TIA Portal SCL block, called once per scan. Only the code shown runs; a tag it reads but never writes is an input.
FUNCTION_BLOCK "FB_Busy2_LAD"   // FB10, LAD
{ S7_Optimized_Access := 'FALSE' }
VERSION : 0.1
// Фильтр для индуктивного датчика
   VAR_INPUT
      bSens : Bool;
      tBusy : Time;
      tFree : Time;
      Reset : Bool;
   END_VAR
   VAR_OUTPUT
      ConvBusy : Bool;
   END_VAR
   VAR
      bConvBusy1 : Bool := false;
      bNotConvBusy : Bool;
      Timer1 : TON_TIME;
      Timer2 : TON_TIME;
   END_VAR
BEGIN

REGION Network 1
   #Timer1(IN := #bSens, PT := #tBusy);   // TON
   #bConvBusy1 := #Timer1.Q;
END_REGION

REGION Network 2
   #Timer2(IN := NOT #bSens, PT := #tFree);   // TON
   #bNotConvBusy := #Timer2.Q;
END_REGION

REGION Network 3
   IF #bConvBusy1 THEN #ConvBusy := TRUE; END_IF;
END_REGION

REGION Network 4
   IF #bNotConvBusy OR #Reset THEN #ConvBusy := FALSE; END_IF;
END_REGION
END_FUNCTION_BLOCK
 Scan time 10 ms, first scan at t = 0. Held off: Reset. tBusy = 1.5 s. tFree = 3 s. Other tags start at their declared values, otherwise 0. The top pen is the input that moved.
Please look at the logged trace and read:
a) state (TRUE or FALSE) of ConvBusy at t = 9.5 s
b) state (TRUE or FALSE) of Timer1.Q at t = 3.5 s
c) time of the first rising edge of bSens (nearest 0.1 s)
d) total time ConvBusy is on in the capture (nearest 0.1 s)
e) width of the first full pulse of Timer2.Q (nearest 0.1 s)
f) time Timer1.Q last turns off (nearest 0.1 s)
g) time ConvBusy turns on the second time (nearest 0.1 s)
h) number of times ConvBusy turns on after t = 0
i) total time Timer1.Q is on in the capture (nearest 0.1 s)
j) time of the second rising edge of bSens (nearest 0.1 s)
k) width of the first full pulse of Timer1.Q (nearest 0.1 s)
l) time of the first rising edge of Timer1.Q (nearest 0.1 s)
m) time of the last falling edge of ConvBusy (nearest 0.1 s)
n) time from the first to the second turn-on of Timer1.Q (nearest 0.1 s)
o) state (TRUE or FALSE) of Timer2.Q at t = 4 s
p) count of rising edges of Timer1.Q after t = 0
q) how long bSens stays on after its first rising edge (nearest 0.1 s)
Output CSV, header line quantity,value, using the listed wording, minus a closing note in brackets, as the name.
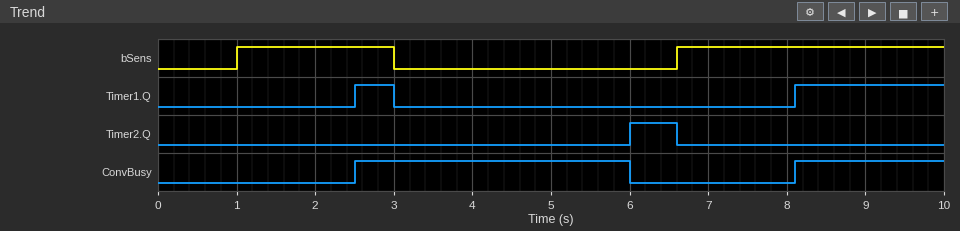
quantity,value
state (TRUE or FALSE) of ConvBusy at t = 9.5 s,TRUE
state (TRUE or FALSE) of Timer1.Q at t = 3.5 s,FALSE
time of the first rising edge of bSens,1.0 s
total time ConvBusy is on in the capture,5.4 s
width of the first full pulse of Timer2.Q,0.6 s
time Timer1.Q last turns off,3.0 s
time ConvBusy turns on the second time,8.1 s
number of times ConvBusy turns on after t = 0,2
total time Timer1.Q is on in the capture,2.4 s
time of the second rising edge of bSens,6.6 s
width of the first full pulse of Timer1.Q,0.5 s
time of the first rising edge of Timer1.Q,2.5 s
time of the last falling edge of ConvBusy,6.0 s
time from the first to the second turn-on of Timer1.Q,5.6 s
state (TRUE or FALSE) of Timer2.Q at t = 4 s,FALSE
count of rising edges of Timer1.Q after t = 0,2
how long bSens stays on after its first rising edge,2.0 s
